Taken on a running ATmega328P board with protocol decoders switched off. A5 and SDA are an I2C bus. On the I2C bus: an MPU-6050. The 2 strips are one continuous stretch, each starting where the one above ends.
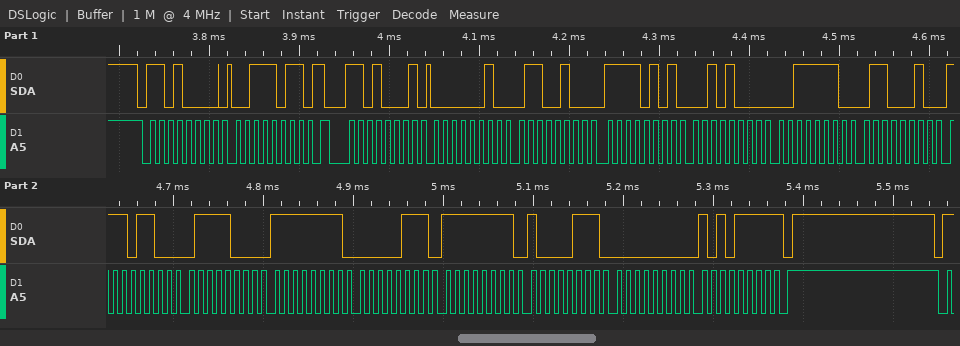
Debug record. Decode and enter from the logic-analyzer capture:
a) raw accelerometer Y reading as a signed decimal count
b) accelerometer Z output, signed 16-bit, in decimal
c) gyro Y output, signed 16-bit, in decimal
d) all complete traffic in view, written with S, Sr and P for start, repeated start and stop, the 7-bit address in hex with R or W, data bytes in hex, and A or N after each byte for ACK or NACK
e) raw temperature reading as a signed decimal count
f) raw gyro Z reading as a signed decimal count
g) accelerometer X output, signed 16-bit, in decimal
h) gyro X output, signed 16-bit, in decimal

-2776
15970
-121
S 68W A 3B A Sr 68R A 02 A 64 A F5 A 28 A 3E A 62 A EC A 78 A FF A 07 A FF A 87 A 00 A AF N P
-5000
175
612
-249
